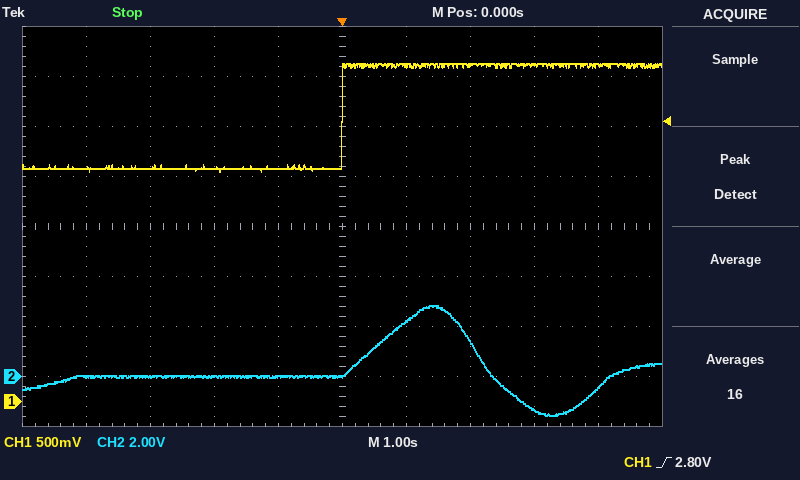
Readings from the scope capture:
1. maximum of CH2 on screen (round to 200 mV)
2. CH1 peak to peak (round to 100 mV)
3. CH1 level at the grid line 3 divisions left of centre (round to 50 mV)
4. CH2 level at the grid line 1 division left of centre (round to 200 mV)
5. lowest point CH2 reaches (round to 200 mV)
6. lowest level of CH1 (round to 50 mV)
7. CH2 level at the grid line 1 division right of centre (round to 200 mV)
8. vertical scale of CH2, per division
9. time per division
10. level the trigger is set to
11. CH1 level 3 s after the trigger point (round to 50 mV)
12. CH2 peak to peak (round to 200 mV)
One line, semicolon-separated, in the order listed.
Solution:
2.8 V; 1.10 V; 2.35 V; 0.0 V; -1.6 V; 2.30 V; 2.2 V; 2 V; 1 s; 2.80 V; 3.35 V; 4.4 V
